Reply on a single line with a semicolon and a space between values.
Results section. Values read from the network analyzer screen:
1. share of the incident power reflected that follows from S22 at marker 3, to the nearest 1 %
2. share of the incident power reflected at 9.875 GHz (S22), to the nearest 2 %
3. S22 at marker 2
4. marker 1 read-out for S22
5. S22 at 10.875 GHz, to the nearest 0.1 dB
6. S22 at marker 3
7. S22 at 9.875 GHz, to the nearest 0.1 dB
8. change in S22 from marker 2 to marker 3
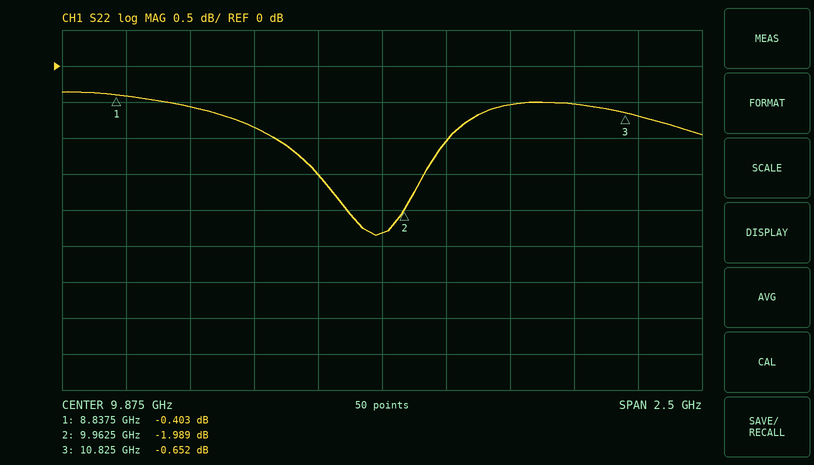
86 %; 58 %; -1.989 dB; -0.403 dB; -0.7 dB; -0.652 dB; -2.3 dB; 1.337 dB
